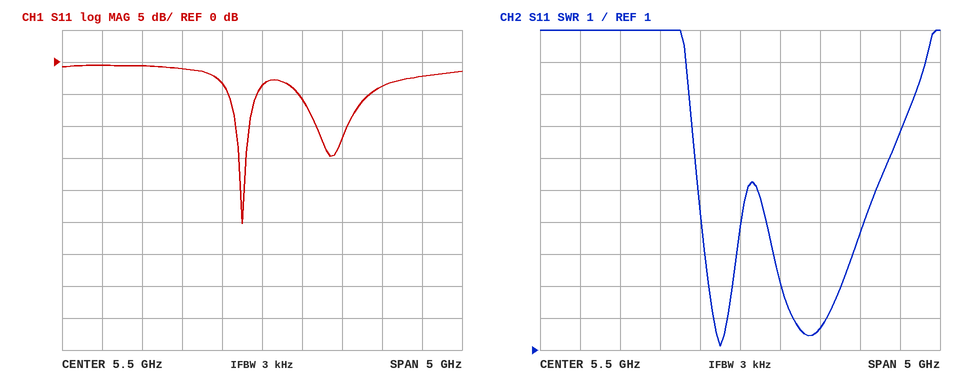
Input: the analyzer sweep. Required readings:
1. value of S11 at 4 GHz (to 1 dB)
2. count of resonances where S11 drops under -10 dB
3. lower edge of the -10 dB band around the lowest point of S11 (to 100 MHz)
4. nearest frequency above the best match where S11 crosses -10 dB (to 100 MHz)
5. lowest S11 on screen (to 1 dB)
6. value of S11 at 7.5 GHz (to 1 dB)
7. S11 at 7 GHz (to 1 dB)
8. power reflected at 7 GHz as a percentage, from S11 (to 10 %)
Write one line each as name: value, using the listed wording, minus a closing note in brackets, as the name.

value of S11 at 4 GHz: -1 dB
count of resonances where S11 drops under -10 dB: 2
lower edge of the -10 dB band around the lowest point of S11: 5.2 GHz
nearest frequency above the best match where S11 crosses -10 dB: 5.3 GHz
lowest S11 on screen: -25 dB
value of S11 at 7.5 GHz: -2 dB
S11 at 7 GHz: -4 dB
power reflected at 7 GHz as a percentage, from S11: 40 %
